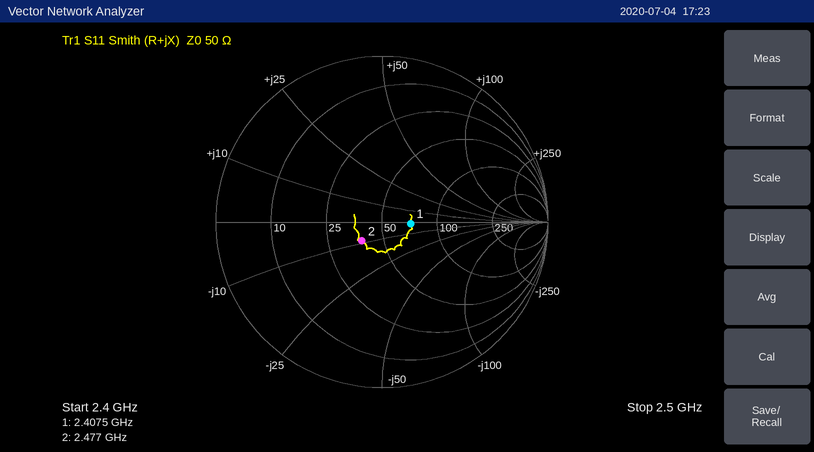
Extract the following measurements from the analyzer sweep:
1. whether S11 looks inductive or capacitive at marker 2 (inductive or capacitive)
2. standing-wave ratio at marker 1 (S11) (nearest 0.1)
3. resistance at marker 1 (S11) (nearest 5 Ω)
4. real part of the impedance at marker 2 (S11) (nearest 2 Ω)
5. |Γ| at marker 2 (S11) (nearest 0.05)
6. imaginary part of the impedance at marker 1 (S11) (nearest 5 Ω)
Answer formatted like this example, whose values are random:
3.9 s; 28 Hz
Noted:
capacitive; 1.4; 70 Ω; 38 Ω; 0.15; 0 Ω
